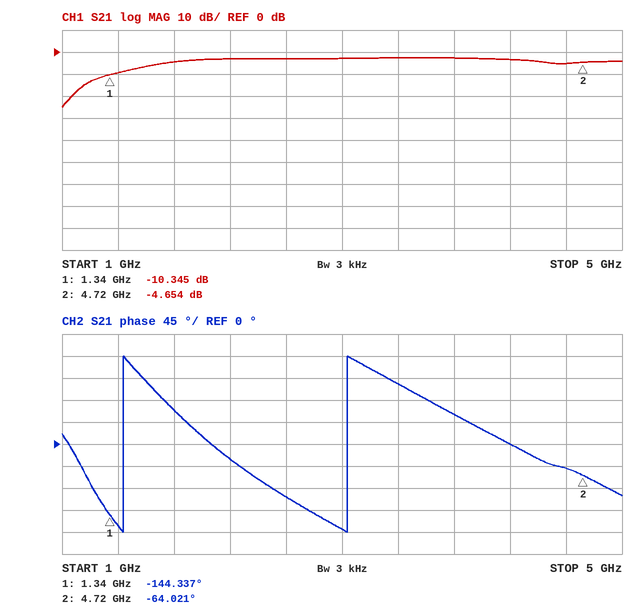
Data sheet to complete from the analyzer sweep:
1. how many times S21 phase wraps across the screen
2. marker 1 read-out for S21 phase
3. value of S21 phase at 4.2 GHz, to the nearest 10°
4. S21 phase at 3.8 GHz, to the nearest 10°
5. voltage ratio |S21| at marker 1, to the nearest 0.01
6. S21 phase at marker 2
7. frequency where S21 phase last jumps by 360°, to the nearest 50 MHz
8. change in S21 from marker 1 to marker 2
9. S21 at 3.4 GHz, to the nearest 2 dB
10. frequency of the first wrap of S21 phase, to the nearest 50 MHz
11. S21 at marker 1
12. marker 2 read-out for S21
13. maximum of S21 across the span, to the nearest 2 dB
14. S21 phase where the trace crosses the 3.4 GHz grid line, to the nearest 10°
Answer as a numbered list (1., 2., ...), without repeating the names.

1. 2
2. -144.337°
3. 0°
4. 60°
5. 0.30
6. -64.021°
7. 3.05 GHz
8. 5.691 dB
9. -2 dB
10. 1.45 GHz
11. -10.345 dB
12. -4.654 dB
13. -2 dB
14. 120°
